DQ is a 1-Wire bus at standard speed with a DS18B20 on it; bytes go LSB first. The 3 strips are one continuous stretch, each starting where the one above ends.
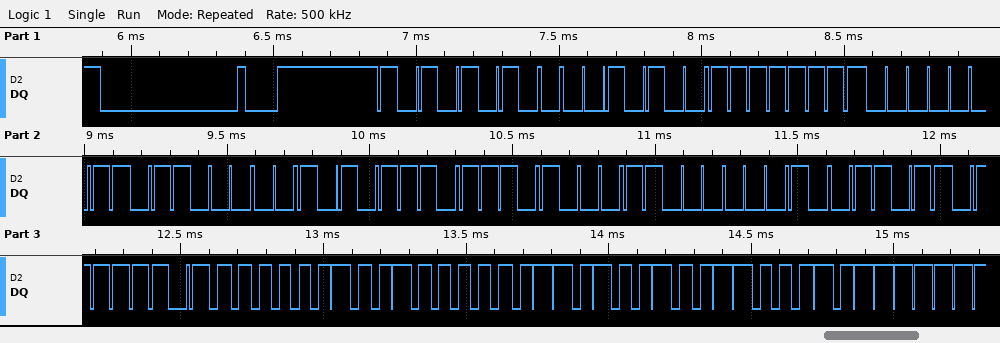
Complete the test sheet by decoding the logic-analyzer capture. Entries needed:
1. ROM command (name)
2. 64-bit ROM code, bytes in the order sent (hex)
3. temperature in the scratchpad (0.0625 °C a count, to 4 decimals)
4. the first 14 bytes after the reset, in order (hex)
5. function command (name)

Match ROM
28 FF C0 06 75 17 03 D9
36.0000 °C
55 28 FF C0 06 75 17 03 D9 BE 40 02 4B 46
Read Scratchpad
